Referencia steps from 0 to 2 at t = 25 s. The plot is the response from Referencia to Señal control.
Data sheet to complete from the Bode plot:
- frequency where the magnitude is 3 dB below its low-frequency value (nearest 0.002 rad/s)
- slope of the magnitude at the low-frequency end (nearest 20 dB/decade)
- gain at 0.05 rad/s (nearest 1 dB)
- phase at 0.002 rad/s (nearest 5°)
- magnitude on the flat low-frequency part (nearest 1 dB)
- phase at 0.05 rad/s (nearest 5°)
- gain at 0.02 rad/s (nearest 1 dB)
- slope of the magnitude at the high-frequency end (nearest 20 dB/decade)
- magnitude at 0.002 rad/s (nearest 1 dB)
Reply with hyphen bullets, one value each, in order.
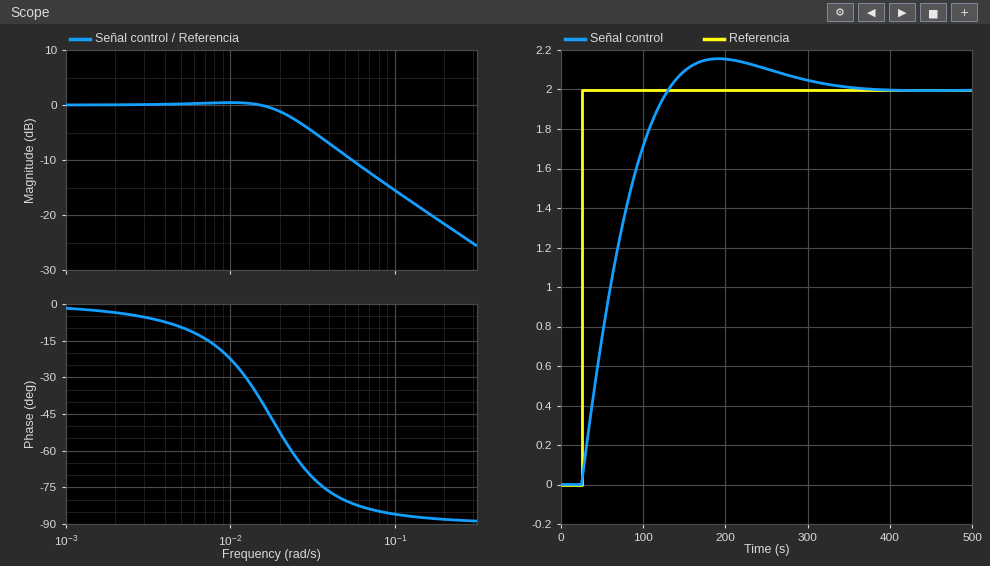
- 0.026 rad/s
- 0 dB/decade
- -9 dB
- -5°
- 0 dB
- -80°
- -1 dB
- -20 dB/decade
- 0 dB
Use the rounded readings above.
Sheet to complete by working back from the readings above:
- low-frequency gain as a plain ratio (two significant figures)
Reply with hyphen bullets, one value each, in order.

- 1.0
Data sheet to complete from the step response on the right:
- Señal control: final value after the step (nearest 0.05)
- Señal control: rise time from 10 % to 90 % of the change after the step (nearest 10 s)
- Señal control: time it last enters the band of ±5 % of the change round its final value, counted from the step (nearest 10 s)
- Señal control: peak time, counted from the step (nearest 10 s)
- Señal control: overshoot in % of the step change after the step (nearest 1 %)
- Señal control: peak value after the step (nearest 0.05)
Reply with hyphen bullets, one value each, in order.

- 2.00
- 80 s
- 230 s
- 170 s
- 8 %
- 2.15
